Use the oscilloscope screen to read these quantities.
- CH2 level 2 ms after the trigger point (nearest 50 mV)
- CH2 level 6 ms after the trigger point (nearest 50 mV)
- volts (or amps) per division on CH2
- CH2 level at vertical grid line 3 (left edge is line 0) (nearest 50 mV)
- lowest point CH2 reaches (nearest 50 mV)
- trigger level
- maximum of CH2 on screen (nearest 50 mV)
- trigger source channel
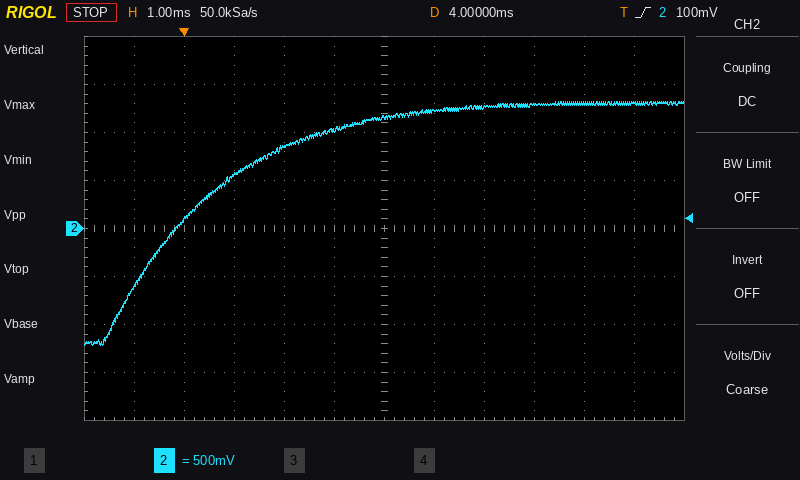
850 mV
1.25 V
500 mV
550 mV
-1.20 V
100 mV
1.30 V
CH2
